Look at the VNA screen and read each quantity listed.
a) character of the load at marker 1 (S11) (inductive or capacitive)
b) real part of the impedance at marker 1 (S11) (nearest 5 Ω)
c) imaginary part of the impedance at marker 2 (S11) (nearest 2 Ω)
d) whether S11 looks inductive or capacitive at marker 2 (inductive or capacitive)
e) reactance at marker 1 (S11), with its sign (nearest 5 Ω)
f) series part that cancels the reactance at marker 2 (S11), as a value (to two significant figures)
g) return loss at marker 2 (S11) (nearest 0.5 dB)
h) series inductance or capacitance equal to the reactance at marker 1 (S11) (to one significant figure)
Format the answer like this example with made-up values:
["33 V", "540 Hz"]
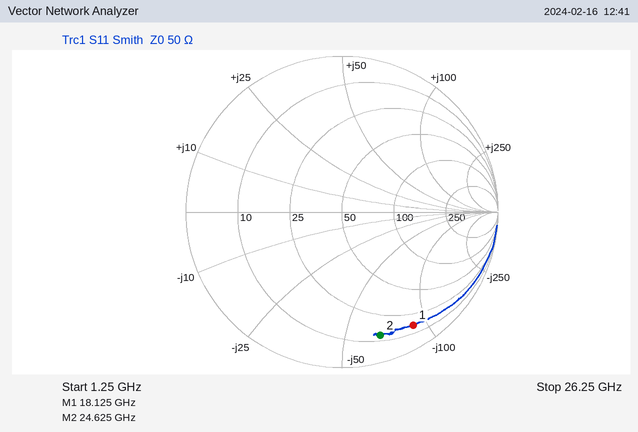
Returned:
["capacitive", "15 Ω", "-66 Ω", "capacitive", "-90 Ω", "430 pH", "1.5 dB", "100 fF"]
